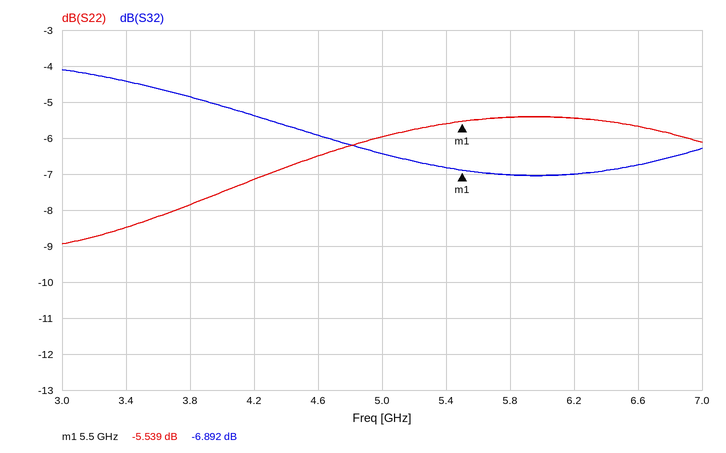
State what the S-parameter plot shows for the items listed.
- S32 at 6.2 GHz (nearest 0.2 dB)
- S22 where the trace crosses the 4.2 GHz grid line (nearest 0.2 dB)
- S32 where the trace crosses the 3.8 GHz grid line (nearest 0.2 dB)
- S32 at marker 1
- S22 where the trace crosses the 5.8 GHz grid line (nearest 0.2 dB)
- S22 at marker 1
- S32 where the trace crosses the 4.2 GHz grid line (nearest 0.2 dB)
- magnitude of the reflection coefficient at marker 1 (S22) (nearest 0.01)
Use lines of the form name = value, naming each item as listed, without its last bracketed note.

S32 at 6.2 GHz = -7.0 dB
S22 where the trace crosses the 4.2 GHz grid line = -7.2 dB
S32 where the trace crosses the 3.8 GHz grid line = -4.8 dB
S32 at marker 1 = -6.892 dB
S22 where the trace crosses the 5.8 GHz grid line = -5.4 dB
S22 at marker 1 = -5.539 dB
S32 where the trace crosses the 4.2 GHz grid line = -5.4 dB
magnitude of the reflection coefficient at marker 1 (S22) = 0.53
